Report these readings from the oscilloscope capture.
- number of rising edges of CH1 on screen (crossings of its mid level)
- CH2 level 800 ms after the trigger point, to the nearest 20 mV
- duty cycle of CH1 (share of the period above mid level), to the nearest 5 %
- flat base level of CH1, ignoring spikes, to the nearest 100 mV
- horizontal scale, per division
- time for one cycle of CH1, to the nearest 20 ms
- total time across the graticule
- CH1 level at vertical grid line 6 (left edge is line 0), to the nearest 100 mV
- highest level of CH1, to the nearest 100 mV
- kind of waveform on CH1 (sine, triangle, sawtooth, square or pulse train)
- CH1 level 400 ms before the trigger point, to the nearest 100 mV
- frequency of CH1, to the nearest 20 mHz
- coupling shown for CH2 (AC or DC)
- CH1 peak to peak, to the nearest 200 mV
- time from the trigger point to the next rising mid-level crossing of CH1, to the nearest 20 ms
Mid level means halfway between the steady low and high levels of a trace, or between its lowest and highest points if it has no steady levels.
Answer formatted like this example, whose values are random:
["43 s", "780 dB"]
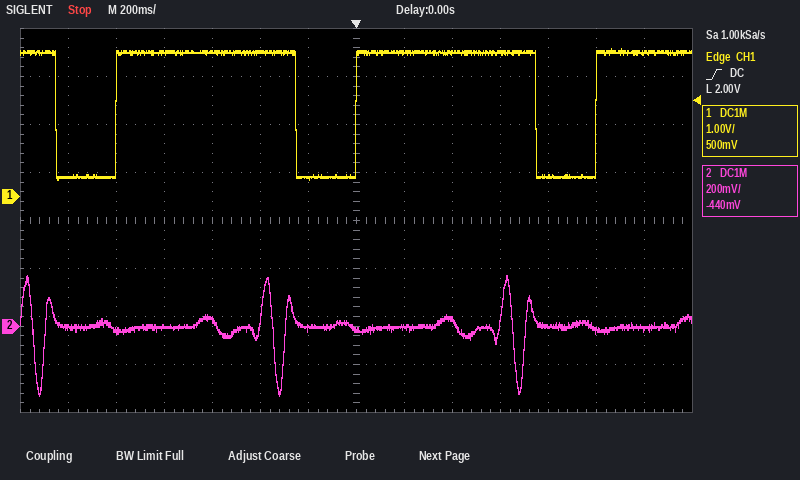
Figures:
["3", "0 mV", "75 %", "400 mV", "200 ms", "1.00 s", "2.8 s", "400 mV", "3.1 V", "pulse train", "3.0 V", "1.00 Hz", "DC", "2.8 V", "1.00 s"]
